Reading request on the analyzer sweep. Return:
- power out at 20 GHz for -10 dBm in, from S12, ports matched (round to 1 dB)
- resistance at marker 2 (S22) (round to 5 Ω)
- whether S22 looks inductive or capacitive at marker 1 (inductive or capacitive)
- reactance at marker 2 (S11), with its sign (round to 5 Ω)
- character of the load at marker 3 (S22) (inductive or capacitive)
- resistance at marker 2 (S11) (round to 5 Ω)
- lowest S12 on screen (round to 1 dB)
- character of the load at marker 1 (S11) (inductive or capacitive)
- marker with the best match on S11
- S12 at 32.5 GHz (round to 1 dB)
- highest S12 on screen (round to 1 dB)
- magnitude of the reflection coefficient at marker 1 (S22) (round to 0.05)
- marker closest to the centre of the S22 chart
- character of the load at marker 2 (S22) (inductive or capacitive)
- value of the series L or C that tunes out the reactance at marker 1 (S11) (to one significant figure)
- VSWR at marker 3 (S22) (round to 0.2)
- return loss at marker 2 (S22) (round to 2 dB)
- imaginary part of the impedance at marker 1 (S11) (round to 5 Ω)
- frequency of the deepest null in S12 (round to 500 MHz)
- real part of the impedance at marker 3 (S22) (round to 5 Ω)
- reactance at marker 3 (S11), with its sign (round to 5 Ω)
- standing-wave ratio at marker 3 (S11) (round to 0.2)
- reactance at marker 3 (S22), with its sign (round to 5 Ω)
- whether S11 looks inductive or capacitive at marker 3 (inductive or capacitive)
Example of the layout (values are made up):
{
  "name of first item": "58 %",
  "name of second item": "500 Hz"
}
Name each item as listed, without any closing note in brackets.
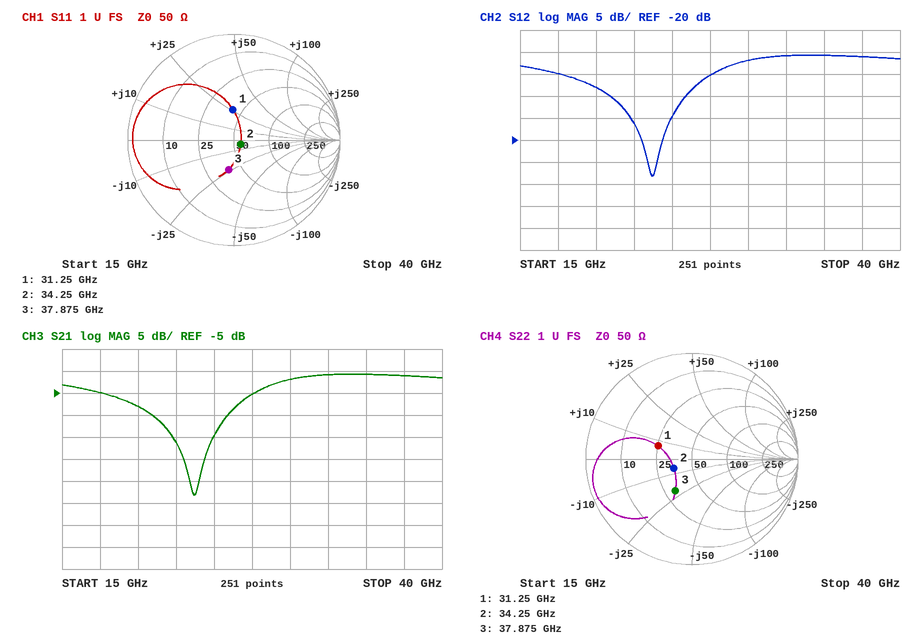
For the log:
{
  "power out at 20 GHz for -10 dBm in, from S12, ports matched": "-18 dBm",
  "resistance at marker 2 (S22)": "35 Ω",
  "whether S22 looks inductive or capacitive at marker 1": "inductive",
  "reactance at marker 2 (S11), with its sign": "-5 Ω",
  "character of the load at marker 3 (S22)": "capacitive",
  "resistance at marker 2 (S11)": "55 Ω",
  "lowest S12 on screen": "-28 dB",
  "character of the load at marker 1 (S11)": "inductive",
  "marker with the best match on S11": "marker 2",
  "S12 at 32.5 GHz": "-1 dB",
  "highest S12 on screen": "-1 dB",
  "magnitude of the reflection coefficient at marker 1 (S22)": "0.35",
  "marker closest to the centre of the S22 chart": "marker 2",
  "character of the load at marker 2 (S22)": "capacitive",
  "value of the series L or C that tunes out the reactance at marker 1 (S11)": "200 fF",
  "VSWR at marker 3 (S22)": "2.0",
  "return loss at marker 2 (S22)": "14 dB",
  "imaginary part of the impedance at marker 1 (S11)": "+25 Ω",
  "frequency of the deepest null in S12": "23.5 GHz",
  "real part of the impedance at marker 3 (S22)": "30 Ω",
  "reactance at marker 3 (S11), with its sign": "-25 Ω",
  "standing-wave ratio at marker 3 (S11)": "1.8",
  "reactance at marker 3 (S22), with its sign": "-20 Ω",
  "whether S11 looks inductive or capacitive at marker 3": "capacitive"
}
